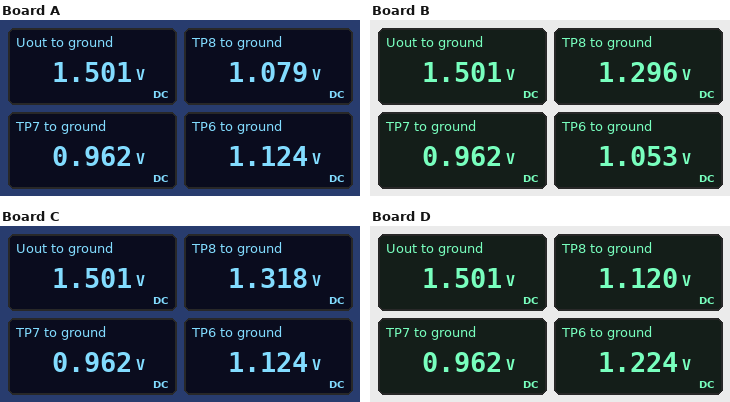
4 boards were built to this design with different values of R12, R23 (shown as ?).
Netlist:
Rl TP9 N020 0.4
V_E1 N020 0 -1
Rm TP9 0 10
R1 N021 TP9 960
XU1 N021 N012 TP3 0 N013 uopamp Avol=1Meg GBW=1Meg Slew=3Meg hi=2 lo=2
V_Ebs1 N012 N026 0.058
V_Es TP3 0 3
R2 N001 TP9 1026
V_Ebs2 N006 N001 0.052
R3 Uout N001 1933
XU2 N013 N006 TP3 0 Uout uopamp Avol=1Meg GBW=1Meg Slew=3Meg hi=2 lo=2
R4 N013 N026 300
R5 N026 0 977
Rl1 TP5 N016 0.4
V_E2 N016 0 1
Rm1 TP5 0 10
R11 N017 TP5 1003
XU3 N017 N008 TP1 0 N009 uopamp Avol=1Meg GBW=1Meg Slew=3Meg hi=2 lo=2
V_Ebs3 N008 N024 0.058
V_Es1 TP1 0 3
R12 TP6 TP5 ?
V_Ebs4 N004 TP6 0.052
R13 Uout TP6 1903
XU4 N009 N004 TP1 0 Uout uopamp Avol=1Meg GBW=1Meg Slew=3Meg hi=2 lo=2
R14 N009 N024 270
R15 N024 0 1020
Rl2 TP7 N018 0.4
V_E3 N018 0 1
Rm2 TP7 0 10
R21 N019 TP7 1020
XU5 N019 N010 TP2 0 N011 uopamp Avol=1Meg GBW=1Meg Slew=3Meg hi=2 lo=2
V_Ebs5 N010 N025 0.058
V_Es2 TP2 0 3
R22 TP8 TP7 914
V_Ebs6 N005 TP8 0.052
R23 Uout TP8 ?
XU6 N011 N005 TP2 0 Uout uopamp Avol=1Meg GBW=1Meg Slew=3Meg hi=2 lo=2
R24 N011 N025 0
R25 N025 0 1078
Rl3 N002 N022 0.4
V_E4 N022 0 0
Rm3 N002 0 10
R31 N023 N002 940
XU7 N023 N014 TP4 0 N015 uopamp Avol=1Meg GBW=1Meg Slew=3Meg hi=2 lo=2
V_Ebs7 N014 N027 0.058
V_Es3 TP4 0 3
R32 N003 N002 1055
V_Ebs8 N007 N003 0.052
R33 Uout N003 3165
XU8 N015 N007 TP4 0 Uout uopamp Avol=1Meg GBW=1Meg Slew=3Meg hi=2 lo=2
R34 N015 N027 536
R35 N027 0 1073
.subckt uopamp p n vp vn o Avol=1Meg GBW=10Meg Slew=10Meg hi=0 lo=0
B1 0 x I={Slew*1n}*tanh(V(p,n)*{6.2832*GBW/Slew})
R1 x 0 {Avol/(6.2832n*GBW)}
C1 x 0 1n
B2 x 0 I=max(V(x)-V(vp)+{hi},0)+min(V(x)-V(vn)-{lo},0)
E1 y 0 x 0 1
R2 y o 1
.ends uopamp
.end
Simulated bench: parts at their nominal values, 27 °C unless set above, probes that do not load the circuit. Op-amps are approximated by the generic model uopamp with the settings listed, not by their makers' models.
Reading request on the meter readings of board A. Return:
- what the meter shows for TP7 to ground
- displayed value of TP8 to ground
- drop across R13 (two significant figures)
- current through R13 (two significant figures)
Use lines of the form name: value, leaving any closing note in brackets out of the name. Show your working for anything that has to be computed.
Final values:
what the meter shows for TP7 to ground: 0.962 V
displayed value of TP8 to ground: 1.079 V
drop across R13: 1.501 V - 1.124 V = 380 mV
current through R13: (1.501 V - 1.124 V) / 1.903 kΩ = 200 µA
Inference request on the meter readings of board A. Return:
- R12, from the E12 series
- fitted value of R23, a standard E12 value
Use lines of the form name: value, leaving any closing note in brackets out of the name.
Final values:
R12, from the E12 series: 820 Ω
fitted value of R23, a standard E12 value: 3.3 kΩ
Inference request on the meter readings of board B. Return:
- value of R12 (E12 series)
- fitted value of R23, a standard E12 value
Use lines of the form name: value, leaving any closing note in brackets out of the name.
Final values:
value of R12: 390 Ω
fitted value of R23, a standard E12 value: 560 Ω
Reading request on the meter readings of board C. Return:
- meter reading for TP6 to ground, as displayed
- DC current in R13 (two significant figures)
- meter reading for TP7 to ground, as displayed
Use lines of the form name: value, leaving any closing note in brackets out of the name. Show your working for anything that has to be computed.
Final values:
meter reading for TP6 to ground, as displayed: 1.124 V
DC current in R13: (1.501 V - 1.124 V) / 1.903 kΩ = 200 µA
meter reading for TP7 to ground, as displayed: 0.962 V
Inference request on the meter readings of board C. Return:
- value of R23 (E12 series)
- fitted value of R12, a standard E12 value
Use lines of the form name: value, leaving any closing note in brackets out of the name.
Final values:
value of R23: 470 Ω
fitted value of R12, a standard E12 value: 820 Ω
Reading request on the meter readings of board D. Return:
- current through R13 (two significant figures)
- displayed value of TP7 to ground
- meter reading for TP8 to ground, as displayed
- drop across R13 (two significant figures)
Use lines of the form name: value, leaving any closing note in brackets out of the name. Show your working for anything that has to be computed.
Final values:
current through R13: (1.501 V - 1.224 V) / 1.903 kΩ = 150 µA
displayed value of TP7 to ground: 0.962 V
meter reading for TP8 to ground, as displayed: 1.120 V
drop across R13: 1.501 V - 1.224 V = 280 mV
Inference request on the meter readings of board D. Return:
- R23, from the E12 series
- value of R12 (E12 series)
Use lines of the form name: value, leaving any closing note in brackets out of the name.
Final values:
R23, from the E12 series: 2.2 kΩ
value of R12: 1.8 kΩ
